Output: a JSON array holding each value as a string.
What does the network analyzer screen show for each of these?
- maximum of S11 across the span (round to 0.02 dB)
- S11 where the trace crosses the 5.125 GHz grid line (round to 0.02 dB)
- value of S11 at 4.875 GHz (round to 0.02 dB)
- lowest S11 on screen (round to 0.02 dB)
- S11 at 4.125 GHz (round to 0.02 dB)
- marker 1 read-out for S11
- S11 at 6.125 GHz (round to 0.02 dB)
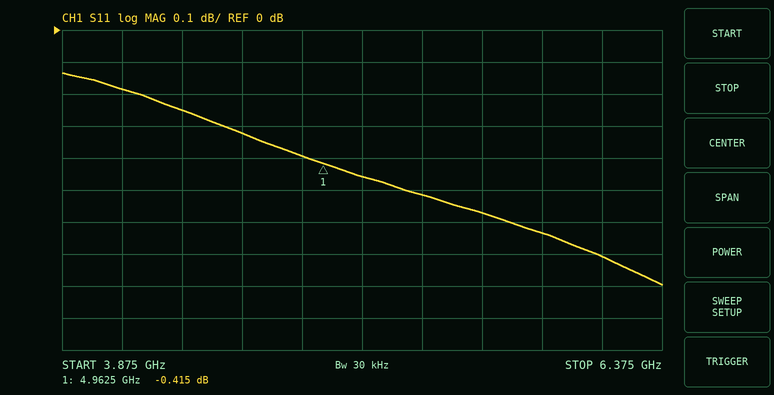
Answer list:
["-0.14 dB", "-0.46 dB", "-0.40 dB", "-0.80 dB", "-0.18 dB", "-0.415 dB", "-0.70 dB"]
